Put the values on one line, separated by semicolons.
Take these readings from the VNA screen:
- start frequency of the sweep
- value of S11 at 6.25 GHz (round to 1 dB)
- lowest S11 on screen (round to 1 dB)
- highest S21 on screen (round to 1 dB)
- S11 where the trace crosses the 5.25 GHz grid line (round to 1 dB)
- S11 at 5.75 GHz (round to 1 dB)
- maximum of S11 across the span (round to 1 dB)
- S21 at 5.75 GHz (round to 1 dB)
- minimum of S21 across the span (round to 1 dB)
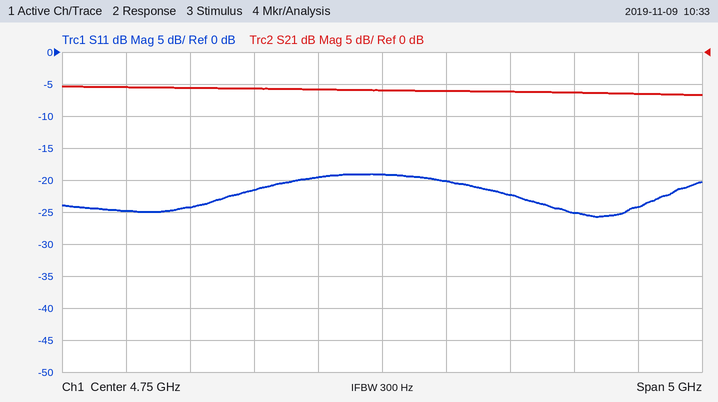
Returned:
2.25 GHz; -25 dB; -26 dB; -5 dB; -20 dB; -22 dB; -19 dB; -6 dB; -7 dB
